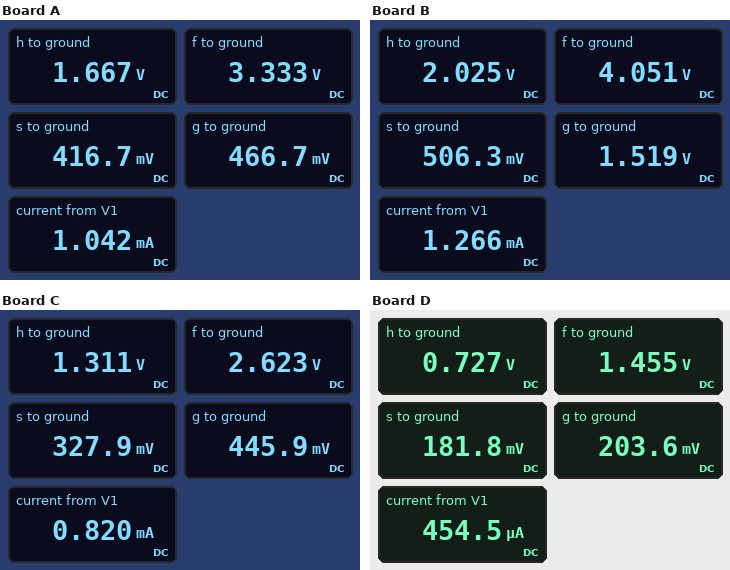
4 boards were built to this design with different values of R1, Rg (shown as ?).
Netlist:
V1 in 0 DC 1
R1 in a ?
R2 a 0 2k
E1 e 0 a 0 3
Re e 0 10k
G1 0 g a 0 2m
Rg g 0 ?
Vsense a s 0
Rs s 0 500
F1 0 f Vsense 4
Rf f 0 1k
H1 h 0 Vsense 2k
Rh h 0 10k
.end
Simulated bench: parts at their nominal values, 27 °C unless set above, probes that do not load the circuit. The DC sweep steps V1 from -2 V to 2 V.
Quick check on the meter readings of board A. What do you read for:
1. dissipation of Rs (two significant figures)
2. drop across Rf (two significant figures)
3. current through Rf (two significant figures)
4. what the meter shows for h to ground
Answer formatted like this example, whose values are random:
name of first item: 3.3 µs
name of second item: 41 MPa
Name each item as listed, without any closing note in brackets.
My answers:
dissipation of Rs: 350 µW
drop across Rf: 3.3 V
current through Rf: 3.3 mA
what the meter shows for h to ground: 1.667 V
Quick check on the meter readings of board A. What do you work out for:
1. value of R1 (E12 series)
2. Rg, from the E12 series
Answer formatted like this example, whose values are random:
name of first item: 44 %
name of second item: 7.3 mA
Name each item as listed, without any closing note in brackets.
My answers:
value of R1: 560 Ω
Rg, from the E12 series: 560 Ω
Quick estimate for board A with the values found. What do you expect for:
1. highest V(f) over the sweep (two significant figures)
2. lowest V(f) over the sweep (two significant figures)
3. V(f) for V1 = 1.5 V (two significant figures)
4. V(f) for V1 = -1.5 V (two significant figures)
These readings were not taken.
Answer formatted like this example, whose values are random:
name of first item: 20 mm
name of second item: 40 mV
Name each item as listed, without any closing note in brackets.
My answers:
highest V(f) over the sweep: 6.7 V
lowest V(f) over the sweep: -6.7 V
V(f) for V1 = 1.5 V: 5.0 V
V(f) for V1 = -1.5 V: -5.0 V
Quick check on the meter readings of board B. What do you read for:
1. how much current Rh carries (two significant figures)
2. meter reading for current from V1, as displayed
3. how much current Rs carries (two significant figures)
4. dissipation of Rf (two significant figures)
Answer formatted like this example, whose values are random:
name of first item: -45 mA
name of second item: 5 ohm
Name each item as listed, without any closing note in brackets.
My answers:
how much current Rh carries: 200 µA
meter reading for current from V1, as displayed: 1.266 mA
how much current Rs carries: 1.0 mA
dissipation of Rf: 16 mW
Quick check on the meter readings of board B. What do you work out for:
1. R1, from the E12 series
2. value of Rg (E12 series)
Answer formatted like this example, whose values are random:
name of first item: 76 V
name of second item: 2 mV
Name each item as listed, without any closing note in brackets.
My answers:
R1, from the E12 series: 390 Ω
value of Rg: 1.5 kΩ
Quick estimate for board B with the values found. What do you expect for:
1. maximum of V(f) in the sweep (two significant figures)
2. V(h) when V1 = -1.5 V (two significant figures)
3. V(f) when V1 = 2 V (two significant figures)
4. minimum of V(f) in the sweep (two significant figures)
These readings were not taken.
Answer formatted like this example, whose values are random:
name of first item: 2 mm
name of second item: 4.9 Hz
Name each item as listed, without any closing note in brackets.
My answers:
maximum of V(f) in the sweep: 8.1 V
V(h) when V1 = -1.5 V: -3.0 V
V(f) when V1 = 2 V: 8.1 V
minimum of V(f) in the sweep: -8.1 V
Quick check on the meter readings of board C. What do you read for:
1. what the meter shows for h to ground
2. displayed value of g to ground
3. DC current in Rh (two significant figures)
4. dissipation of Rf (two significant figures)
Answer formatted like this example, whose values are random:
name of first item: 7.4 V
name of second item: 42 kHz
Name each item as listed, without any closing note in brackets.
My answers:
what the meter shows for h to ground: 1.311 V
displayed value of g to ground: 445.9 mV
DC current in Rh: 130 µA
dissipation of Rf: 6.9 mW
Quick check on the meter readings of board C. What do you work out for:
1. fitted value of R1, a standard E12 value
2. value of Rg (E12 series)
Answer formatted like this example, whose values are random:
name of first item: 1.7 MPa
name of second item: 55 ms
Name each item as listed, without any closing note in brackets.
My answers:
fitted value of R1, a standard E12 value: 820 Ω
value of Rg: 680 Ω
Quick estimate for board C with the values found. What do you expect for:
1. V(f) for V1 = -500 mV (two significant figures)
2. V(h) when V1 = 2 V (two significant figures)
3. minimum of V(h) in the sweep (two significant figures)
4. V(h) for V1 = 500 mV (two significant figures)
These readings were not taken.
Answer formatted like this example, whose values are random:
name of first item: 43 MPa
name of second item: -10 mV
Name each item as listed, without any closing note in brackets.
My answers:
V(f) for V1 = -500 mV: -1.3 V
V(h) when V1 = 2 V: 2.6 V
minimum of V(h) in the sweep: -2.6 V
V(h) for V1 = 500 mV: 660 mV
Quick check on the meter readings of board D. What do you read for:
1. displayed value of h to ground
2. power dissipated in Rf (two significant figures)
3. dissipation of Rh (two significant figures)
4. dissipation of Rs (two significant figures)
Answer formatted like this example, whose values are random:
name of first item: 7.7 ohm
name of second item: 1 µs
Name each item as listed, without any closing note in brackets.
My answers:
displayed value of h to ground: 0.727 V
power dissipated in Rf: 2.1 mW
dissipation of Rh: 53 µW
dissipation of Rs: 66 µW
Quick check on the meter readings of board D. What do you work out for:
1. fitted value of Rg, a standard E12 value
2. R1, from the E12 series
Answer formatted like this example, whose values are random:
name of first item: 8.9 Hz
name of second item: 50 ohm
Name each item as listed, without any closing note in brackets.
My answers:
fitted value of Rg, a standard E12 value: 560 Ω
R1, from the E12 series: 1.8 kΩ
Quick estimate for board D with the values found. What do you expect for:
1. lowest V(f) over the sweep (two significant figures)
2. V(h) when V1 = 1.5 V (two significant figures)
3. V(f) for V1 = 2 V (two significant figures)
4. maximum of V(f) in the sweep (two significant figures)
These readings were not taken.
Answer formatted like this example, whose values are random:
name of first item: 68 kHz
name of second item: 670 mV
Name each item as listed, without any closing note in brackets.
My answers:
lowest V(f) over the sweep: -2.9 V
V(h) when V1 = 1.5 V: 1.1 V
V(f) for V1 = 2 V: 2.9 V
maximum of V(f) in the sweep: 2.9 V
